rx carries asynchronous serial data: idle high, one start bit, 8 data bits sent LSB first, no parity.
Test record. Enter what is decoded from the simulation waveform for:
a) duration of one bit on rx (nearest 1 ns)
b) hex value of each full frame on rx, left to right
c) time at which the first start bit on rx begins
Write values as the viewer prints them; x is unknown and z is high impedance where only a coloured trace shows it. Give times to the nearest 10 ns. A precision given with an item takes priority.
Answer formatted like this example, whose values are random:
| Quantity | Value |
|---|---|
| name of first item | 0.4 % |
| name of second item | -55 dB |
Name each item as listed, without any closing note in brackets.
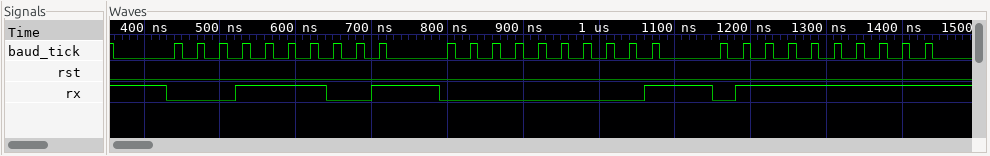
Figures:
| Quantity | Value |
|---|---|
| duration of one bit on rx | 30 ns |
| hex value of each full frame on rx, left to right | 3C, 00, FF |
| time at which the first start bit on rx begins | 430 ns |
